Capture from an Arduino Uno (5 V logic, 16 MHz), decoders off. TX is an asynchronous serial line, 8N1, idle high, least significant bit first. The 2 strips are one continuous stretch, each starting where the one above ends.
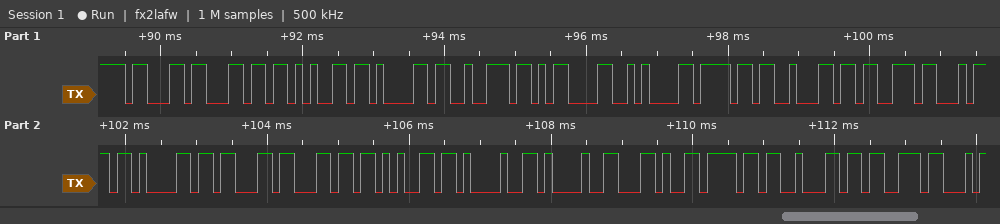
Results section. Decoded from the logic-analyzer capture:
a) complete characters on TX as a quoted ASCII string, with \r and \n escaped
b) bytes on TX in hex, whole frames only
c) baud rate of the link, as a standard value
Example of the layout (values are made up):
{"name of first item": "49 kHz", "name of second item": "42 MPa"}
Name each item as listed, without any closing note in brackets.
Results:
{"complete characters on TX as a quoted ASCII string, with \\r and \\n escaped": "\"clear\\r\\nobstacle!!,obs\"", "bytes on TX in hex, whole frames only": "63 6C 65 61 72 0D 0A 6F 62 73 74 61 63 6C 65 21 21 2C 6F 62 73", "baud rate of the link, as a standard value": "9600 baud"}
